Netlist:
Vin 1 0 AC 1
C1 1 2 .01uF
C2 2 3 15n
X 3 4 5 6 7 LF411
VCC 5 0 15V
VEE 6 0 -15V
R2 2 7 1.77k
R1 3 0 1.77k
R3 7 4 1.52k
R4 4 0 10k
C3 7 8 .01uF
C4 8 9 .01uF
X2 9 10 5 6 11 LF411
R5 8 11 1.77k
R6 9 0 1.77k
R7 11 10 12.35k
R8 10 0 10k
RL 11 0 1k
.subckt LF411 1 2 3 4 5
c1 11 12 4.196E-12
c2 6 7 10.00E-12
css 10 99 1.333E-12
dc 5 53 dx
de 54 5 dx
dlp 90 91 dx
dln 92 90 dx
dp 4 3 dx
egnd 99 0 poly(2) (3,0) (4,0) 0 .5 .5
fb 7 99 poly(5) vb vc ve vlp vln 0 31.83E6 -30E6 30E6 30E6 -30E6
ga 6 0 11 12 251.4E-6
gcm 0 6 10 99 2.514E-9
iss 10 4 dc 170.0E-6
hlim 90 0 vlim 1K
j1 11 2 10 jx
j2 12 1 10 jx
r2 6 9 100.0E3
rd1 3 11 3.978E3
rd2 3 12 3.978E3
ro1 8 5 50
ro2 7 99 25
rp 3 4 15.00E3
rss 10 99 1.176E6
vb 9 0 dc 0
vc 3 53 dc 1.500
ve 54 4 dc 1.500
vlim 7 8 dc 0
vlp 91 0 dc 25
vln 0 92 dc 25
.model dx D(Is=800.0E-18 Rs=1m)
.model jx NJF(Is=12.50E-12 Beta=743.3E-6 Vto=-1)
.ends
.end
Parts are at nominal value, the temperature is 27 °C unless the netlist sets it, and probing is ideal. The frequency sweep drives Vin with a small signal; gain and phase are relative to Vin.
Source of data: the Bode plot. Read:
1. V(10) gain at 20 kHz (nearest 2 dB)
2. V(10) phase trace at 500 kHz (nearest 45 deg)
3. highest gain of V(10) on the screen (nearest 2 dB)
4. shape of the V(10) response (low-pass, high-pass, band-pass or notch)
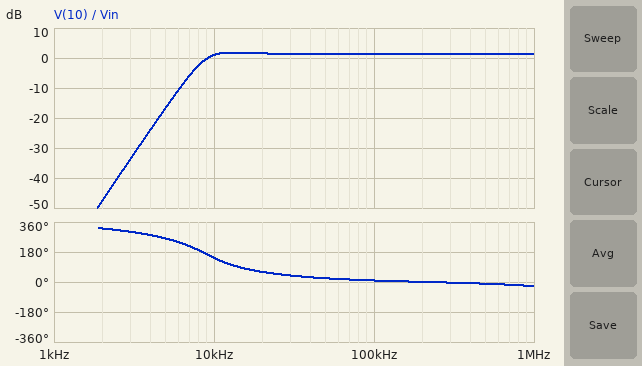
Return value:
2 dB
0 deg
2 dB
high-pass
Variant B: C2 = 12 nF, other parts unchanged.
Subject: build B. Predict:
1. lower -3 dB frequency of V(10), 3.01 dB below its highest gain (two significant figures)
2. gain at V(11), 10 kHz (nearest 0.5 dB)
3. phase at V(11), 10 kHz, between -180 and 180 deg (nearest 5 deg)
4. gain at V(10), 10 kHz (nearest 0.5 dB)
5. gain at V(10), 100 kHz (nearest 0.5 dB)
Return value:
9.5 kHz
7.5 dB
150 deg
0.5 dB
1.0 dB
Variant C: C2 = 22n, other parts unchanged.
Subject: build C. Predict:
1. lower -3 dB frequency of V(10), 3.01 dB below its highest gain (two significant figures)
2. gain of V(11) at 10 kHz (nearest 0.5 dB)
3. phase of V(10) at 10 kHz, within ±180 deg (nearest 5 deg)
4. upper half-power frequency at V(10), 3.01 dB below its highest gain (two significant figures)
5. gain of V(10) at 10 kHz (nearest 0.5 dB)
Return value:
8.5 kHz
8.5 dB
135 deg
4.8 MHz
1.5 dB
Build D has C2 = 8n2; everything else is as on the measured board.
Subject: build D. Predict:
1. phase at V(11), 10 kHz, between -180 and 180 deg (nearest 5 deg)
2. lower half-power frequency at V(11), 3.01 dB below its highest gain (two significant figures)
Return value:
165 deg
11 kHz
